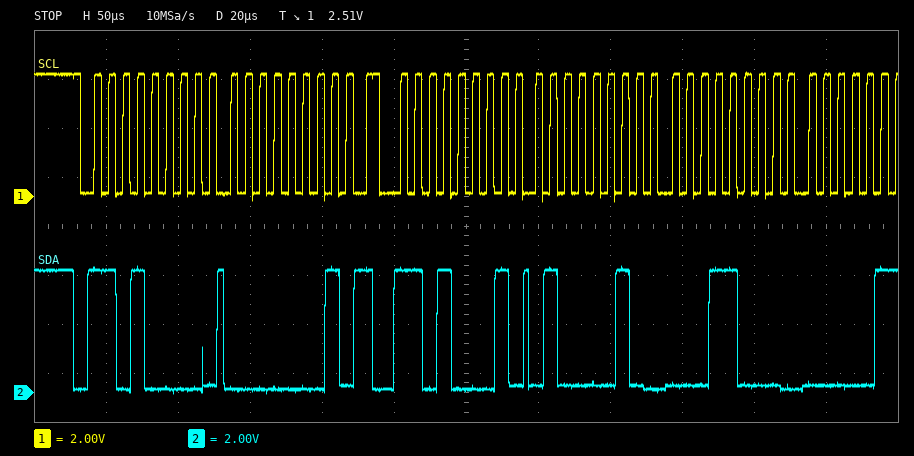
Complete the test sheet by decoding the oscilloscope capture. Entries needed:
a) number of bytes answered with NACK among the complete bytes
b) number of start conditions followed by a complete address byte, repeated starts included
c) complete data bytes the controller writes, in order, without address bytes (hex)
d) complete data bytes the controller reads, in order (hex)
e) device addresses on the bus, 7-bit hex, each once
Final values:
0
2
01
42 18
0x68
